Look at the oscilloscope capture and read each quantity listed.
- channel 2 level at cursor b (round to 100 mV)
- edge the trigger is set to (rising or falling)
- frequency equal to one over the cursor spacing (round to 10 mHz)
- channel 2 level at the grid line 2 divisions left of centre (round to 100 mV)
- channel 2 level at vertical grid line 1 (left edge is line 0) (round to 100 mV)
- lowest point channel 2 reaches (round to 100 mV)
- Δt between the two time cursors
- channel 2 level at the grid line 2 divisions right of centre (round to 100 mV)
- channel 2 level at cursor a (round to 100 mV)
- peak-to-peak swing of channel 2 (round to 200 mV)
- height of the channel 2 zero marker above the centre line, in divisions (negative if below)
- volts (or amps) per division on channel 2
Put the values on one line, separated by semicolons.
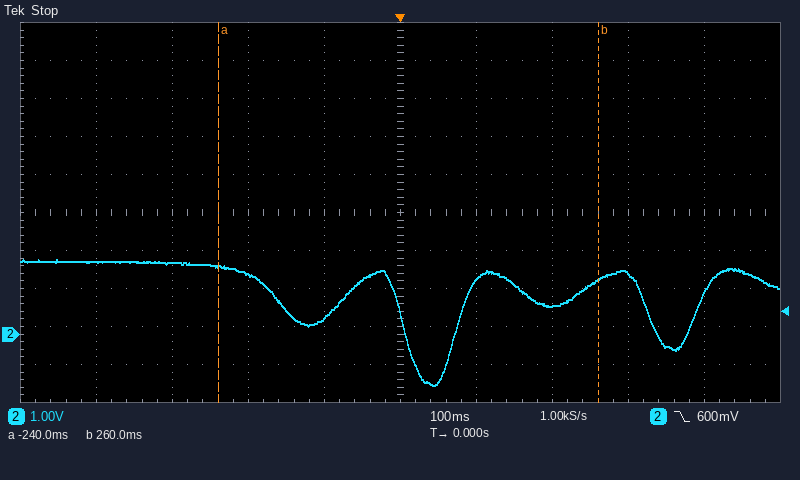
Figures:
1.4 V; falling; 2.00 Hz; 1.6 V; 1.9 V; -1.4 V; 500 ms; 700 mV; 1.8 V; 3.4 V; -3.2 div; 1 V
